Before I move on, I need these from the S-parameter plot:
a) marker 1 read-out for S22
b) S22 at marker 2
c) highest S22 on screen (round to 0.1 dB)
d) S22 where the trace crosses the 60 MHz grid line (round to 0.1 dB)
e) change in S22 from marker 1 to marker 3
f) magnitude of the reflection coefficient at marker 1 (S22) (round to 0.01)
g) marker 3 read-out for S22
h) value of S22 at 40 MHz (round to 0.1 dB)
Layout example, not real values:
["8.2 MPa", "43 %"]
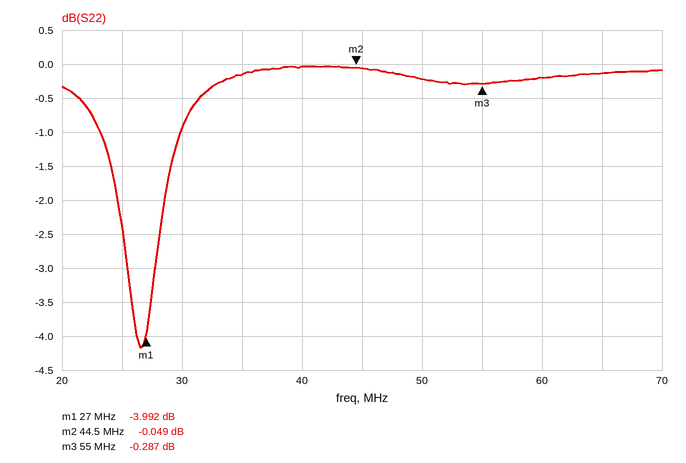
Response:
["-3.992 dB", "-0.049 dB", "0.0 dB", "-0.2 dB", "3.705 dB", "0.63", "-0.287 dB", "0.0 dB"]
